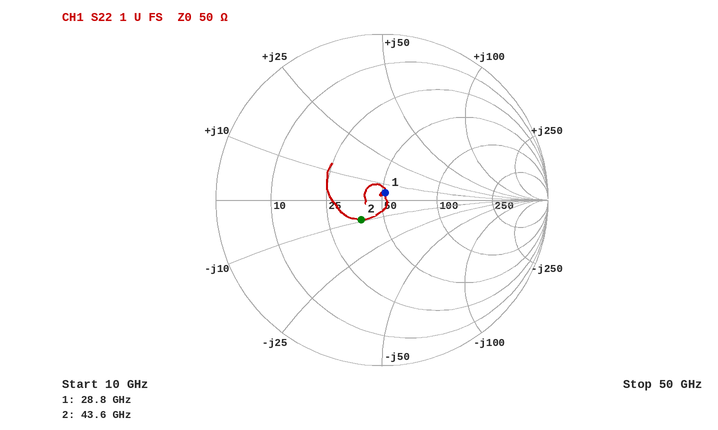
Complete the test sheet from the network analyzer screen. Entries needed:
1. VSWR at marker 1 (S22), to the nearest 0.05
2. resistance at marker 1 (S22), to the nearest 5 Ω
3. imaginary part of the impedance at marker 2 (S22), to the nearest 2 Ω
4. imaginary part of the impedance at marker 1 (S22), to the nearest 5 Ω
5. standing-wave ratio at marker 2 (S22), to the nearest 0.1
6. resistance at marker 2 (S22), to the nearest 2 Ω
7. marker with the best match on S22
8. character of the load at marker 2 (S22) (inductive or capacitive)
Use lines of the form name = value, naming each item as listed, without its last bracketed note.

VSWR at marker 1 (S22), to the nearest 0.05 = 1.10
resistance at marker 1 (S22), to the nearest 5 Ω = 50 Ω
imaginary part of the impedance at marker 2 (S22), to the nearest 2 Ω = -10 Ω
imaginary part of the impedance at marker 1 (S22), to the nearest 5 Ω = +5 Ω
standing-wave ratio at marker 2 (S22), to the nearest 0.1 = 1.4
resistance at marker 2 (S22), to the nearest 2 Ω = 38 Ω
marker with the best match on S22 = marker 1
character of the load at marker 2 (S22) = capacitive
